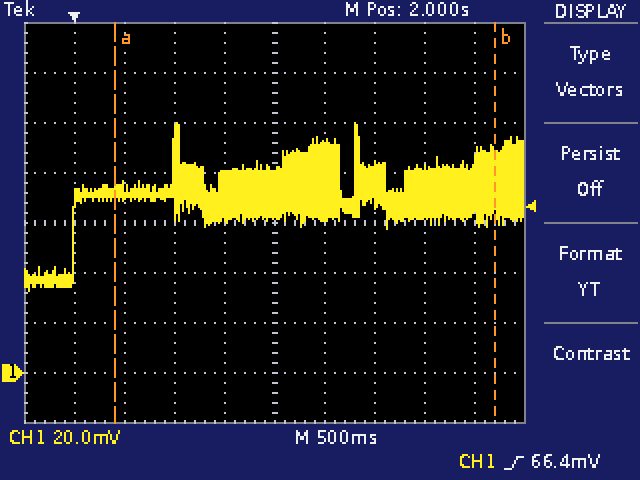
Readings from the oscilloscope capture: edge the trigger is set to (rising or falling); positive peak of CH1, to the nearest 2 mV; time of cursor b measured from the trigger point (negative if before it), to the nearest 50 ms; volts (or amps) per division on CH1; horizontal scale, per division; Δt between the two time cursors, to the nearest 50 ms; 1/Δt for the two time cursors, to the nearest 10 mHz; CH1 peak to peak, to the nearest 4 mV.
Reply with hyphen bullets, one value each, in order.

- rising
- 100 mV
- +4.20 s
- 20 mV
- 500 ms
- 3.80 s
- 260 mHz
- 68 mV
